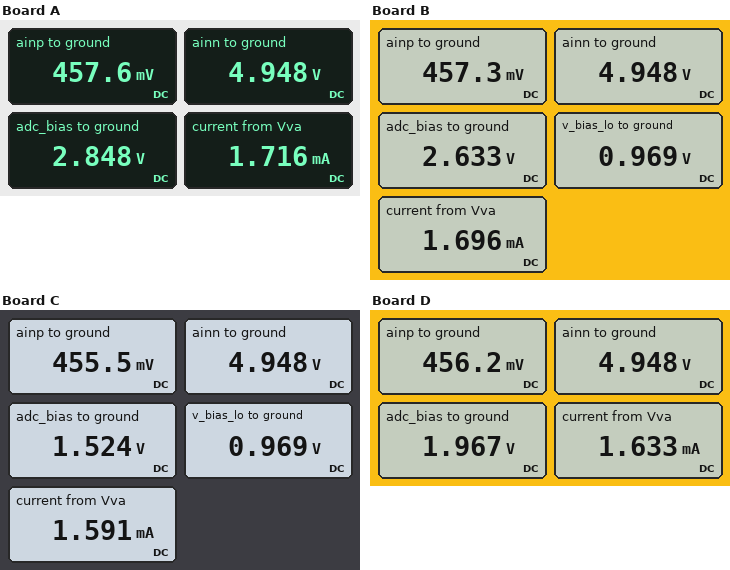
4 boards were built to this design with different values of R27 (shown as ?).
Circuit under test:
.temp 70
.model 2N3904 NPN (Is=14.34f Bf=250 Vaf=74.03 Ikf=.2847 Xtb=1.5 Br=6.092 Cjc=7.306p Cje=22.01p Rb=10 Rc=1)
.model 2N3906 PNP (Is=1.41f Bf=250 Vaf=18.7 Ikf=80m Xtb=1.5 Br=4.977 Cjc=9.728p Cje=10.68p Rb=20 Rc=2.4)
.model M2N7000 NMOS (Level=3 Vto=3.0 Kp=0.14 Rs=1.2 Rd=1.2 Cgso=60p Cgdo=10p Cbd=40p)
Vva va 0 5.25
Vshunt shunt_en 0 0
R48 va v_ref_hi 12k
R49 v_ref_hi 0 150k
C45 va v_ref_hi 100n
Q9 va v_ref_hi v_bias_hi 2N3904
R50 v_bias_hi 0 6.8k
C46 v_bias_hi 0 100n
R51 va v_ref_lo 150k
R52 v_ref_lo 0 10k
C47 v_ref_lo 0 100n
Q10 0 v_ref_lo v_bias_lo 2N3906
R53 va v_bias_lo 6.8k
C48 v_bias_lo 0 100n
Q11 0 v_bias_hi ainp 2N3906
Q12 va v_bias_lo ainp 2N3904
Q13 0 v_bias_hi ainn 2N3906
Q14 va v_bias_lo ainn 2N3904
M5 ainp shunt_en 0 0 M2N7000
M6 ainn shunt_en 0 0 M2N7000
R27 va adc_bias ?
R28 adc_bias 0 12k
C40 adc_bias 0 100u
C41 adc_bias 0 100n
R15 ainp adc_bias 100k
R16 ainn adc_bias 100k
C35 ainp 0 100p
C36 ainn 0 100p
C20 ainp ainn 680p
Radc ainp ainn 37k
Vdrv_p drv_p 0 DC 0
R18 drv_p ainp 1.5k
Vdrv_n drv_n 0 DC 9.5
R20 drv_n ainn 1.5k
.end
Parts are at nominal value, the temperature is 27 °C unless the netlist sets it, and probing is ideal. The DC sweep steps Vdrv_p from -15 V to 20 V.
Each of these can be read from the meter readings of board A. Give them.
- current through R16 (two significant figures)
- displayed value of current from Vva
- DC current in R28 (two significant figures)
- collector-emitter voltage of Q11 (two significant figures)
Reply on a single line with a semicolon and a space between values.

21 µA; 1.716 mA; 240 µA; -460 mV
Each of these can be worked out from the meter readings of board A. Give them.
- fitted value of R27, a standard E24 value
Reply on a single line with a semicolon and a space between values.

10 kΩ
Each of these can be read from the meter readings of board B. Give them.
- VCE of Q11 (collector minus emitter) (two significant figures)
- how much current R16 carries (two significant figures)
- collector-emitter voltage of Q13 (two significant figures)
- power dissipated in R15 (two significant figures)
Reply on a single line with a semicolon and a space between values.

-460 mV; 23 µA; -4.9 V; 47 µW
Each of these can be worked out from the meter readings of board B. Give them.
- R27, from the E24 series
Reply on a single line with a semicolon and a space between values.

12 kΩ
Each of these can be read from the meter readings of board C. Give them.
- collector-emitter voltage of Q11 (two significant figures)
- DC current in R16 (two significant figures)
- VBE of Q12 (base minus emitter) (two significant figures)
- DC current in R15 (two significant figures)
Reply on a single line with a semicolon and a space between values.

-460 mV; 34 µA; 510 mV; 11 µA
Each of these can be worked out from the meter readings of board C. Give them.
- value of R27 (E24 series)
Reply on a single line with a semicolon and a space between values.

36 kΩ
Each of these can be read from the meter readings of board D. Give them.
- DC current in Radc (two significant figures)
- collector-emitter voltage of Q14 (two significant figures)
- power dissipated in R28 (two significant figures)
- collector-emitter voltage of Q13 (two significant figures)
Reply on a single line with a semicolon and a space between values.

120 µA; 300 mV; 320 µW; -4.9 V
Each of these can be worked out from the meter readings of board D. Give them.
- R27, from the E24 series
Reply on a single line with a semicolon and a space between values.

22 kΩ
